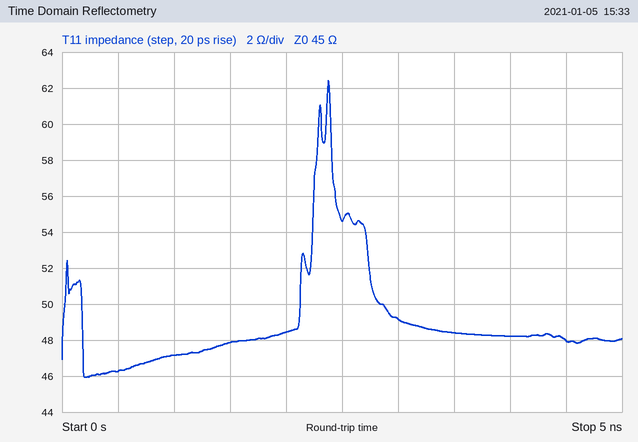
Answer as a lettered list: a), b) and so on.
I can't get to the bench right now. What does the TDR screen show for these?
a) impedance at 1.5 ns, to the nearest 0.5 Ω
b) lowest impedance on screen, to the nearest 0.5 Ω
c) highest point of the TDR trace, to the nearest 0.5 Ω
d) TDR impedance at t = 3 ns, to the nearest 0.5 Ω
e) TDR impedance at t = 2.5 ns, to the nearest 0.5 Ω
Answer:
a) 48.0 Ω
b) 46.0 Ω
c) 62.5 Ω
d) 49.0 Ω
e) 54.5 Ω
